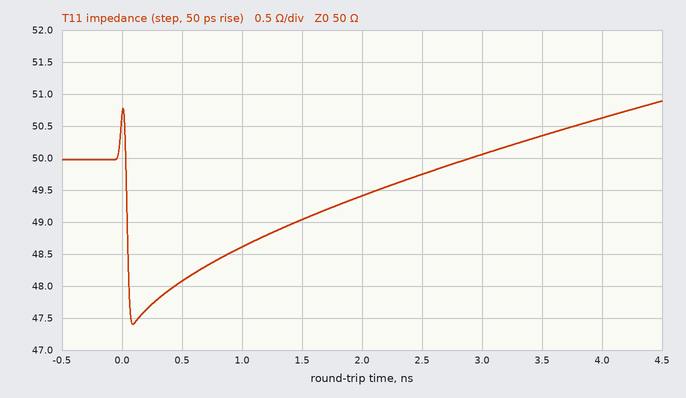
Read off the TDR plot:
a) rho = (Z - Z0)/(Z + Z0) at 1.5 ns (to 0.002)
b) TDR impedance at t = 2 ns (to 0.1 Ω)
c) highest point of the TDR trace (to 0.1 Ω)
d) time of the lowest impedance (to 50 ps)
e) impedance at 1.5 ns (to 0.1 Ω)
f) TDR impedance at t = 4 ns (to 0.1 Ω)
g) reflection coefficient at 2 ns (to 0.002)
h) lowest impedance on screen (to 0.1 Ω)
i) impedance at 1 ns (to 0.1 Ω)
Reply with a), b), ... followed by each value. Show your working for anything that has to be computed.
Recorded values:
a) (49 − 50)/(49 + 50) ≈ -0.010
b) 49.4 Ω
c) 50.9 Ω
d) 100 ps
e) 49.0 Ω
f) 50.6 Ω
g) (49.4 − 50)/(49.4 + 50) ≈ -0.006
h) 47.4 Ω
i) 48.6 Ω
